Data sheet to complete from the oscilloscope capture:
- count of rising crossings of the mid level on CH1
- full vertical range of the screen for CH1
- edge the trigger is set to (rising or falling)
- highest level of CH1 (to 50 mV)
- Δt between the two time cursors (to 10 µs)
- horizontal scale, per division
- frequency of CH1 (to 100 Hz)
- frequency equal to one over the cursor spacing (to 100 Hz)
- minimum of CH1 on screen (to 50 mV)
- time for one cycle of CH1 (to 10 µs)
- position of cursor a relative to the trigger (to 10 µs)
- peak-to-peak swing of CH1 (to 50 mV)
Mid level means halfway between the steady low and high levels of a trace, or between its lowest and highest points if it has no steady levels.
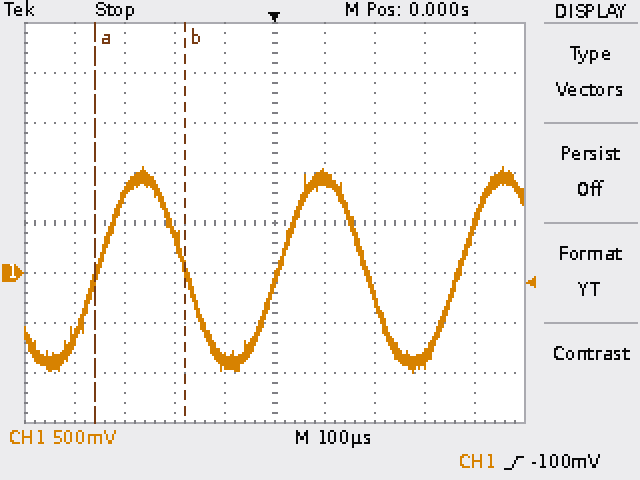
3
4 V
rising
1.05 V
180 µs
100 µs
2.8 kHz
5.6 kHz
-1.00 V
360 µs
-360 µs
2.05 V
